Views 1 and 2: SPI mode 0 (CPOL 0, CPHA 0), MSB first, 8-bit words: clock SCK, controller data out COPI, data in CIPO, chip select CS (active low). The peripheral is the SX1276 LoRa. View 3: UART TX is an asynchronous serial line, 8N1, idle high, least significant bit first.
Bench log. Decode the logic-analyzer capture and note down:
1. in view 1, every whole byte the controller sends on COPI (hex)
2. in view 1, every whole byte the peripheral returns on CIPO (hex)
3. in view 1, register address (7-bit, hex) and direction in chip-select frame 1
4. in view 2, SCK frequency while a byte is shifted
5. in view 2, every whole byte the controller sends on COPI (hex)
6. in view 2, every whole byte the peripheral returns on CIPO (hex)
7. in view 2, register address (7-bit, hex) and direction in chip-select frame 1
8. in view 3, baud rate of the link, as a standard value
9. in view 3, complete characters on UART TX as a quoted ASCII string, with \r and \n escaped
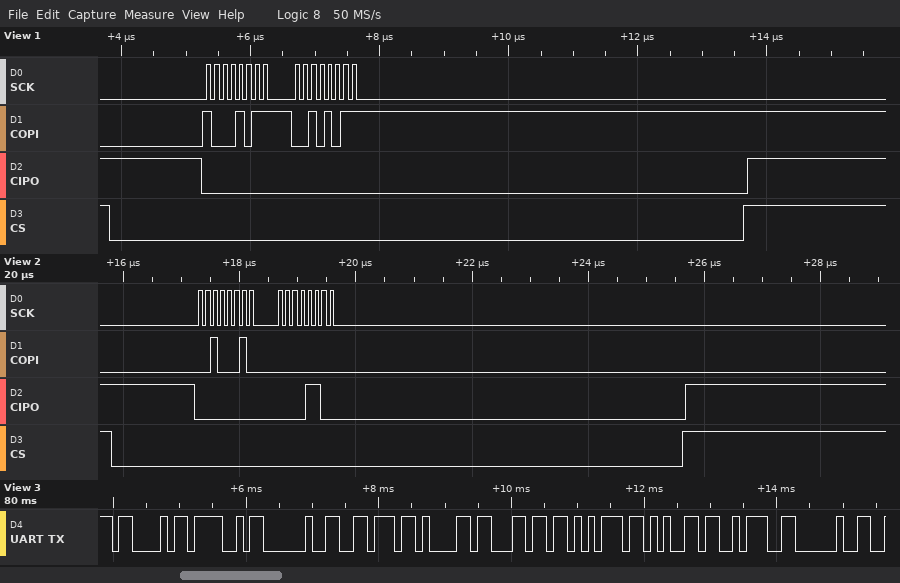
0x8B 0x2B
0x00 0x00
0x0B write
8 MHz
0x22 0x00
0x00 0x0C
0x22 read
9600 baud
"CO value: "
